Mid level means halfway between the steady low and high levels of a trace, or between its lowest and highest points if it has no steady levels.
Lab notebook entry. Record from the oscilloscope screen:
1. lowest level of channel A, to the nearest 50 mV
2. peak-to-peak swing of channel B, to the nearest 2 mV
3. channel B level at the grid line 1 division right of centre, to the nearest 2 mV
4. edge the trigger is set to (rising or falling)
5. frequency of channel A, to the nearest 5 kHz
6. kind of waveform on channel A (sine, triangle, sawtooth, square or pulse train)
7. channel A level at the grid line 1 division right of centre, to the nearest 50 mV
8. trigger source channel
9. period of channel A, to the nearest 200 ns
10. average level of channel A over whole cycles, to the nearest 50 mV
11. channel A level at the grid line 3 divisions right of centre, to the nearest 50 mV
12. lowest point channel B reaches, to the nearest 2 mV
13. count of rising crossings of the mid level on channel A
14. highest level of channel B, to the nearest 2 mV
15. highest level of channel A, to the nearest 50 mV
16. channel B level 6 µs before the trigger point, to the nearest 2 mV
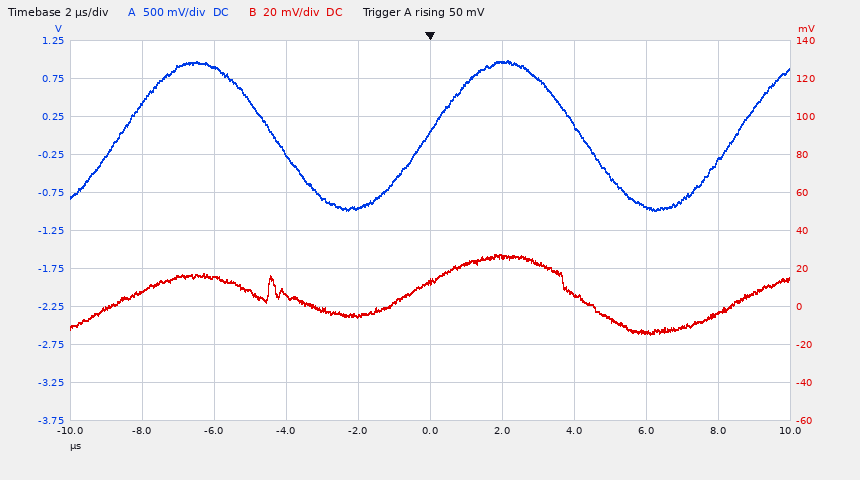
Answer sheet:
-1.00 V
42 mV
26 mV
rising
115 kHz
sine
950 mV
channel A
8.6 µs
0 mV
-950 mV
-14 mV
3
28 mV
1.00 V
16 mV
